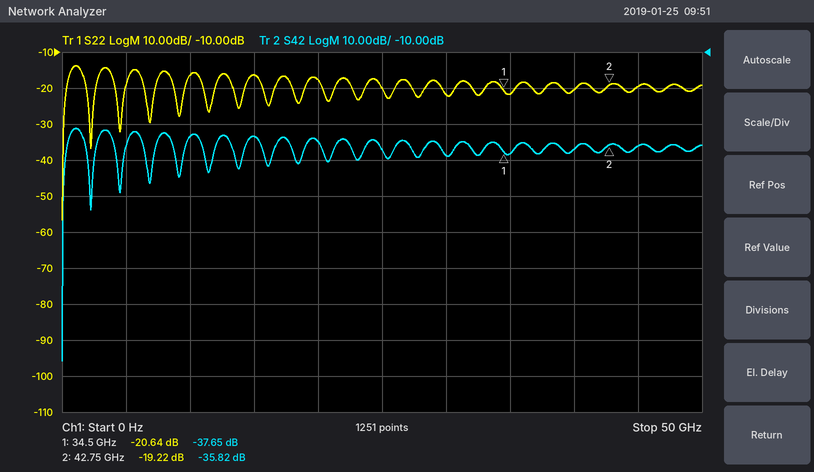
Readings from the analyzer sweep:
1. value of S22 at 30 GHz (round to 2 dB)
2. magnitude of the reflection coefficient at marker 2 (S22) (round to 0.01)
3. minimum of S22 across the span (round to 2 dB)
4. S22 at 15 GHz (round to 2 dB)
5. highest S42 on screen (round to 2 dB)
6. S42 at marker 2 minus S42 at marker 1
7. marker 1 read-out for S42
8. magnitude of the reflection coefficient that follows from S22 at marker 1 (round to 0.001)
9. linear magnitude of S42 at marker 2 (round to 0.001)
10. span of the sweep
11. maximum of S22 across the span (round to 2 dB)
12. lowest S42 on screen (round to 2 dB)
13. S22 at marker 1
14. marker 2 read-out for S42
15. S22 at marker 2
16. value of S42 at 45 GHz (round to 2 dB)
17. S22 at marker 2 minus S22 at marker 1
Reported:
-22 dB
0.11
-56 dB
-16 dB
-32 dB
1.83 dB
-37.65 dB
0.093
0.016
50 GHz
-14 dB
-96 dB
-20.64 dB
-35.82 dB
-19.22 dB
-36 dB
1.42 dB
